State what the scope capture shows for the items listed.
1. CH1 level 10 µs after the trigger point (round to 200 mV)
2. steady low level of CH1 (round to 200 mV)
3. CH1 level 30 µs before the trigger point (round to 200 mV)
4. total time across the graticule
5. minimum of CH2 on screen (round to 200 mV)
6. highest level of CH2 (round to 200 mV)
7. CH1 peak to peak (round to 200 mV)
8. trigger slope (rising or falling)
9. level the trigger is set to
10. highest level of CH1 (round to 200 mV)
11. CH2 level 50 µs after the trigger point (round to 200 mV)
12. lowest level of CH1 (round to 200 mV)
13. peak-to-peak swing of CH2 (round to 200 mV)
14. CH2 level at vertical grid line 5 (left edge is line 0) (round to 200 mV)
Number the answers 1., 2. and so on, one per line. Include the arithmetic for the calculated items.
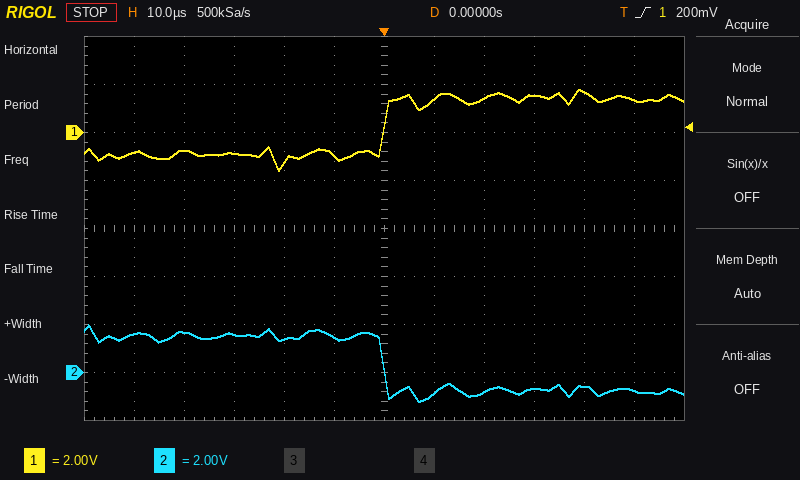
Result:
1. 1.4 V
2. -1.0 V
3. -800 mV
4. 120 µs
5. -1.2 V
6. 2.0 V
7. 1.8 V − (-1.6 V) = 3.4 V
8. rising
9. 200 mV
10. 1.8 V
11. -800 mV
12. -1.6 V
13. 2.0 V − (-1.2 V) = 3.2 V
14. 1.4 V
